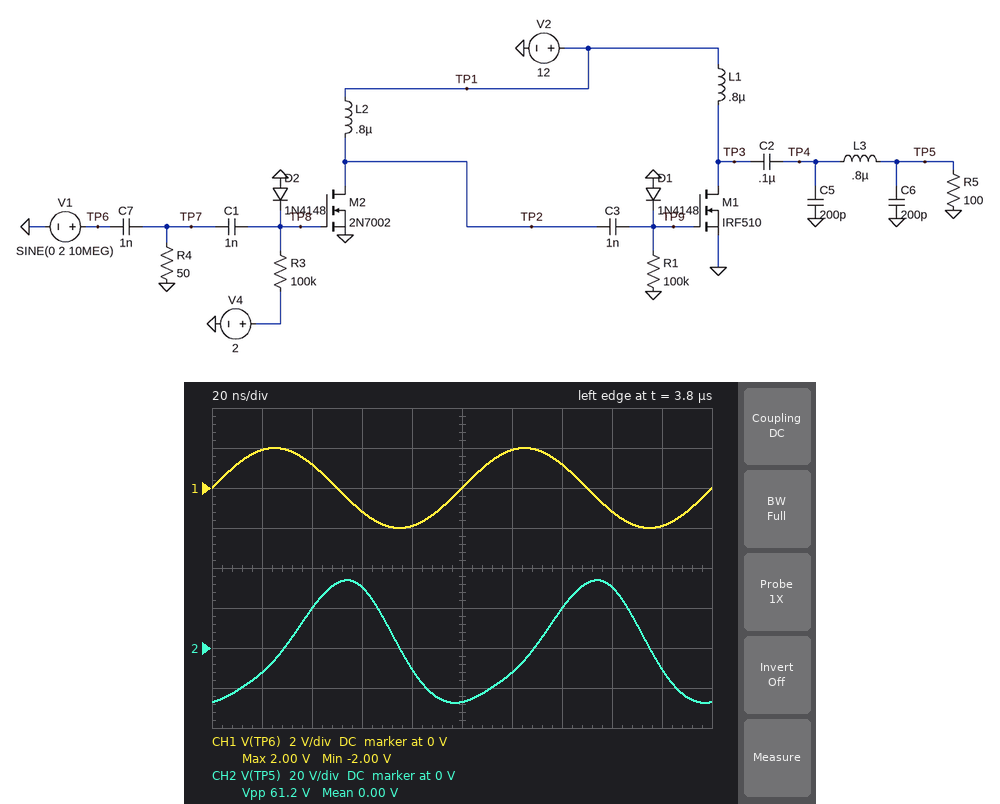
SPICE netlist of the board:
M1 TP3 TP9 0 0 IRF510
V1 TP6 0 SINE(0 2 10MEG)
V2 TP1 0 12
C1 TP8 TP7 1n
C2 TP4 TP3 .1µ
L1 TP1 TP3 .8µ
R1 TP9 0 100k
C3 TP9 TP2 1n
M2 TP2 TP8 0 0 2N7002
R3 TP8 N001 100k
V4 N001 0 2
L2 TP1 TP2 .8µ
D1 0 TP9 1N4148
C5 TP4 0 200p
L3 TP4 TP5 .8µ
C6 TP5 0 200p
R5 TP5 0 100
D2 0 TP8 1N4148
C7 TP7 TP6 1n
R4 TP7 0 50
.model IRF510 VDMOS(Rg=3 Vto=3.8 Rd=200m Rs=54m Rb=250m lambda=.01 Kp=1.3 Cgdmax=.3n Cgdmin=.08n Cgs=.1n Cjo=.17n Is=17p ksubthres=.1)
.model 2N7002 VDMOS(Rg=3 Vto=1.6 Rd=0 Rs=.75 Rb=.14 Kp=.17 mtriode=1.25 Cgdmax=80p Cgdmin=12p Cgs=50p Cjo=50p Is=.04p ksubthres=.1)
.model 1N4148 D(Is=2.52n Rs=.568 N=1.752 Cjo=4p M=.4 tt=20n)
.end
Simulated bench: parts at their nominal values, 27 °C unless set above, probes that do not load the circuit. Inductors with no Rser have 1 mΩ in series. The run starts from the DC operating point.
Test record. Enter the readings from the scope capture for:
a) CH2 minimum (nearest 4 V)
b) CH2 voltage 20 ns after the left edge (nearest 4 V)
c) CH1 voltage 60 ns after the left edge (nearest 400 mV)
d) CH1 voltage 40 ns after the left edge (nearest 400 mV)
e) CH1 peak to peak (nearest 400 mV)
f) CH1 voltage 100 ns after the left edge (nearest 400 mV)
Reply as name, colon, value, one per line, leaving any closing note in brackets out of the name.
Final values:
CH2 minimum: -28 V
CH2 voltage 20 ns after the left edge: -12 V
CH1 voltage 60 ns after the left edge: -1.2 V
CH1 voltage 40 ns after the left edge: 1.2 V
CH1 peak to peak: 4.0 V
CH1 voltage 100 ns after the left edge: 0 V
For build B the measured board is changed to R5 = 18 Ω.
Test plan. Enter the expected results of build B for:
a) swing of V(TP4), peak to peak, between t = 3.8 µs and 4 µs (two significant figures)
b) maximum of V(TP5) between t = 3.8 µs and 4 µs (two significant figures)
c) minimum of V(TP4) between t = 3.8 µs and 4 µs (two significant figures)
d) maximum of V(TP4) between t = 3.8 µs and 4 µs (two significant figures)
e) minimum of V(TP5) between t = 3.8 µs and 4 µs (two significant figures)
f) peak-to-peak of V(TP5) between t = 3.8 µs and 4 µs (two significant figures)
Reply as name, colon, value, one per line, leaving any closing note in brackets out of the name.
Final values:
swing of V(TP4), peak to peak, between t = 3.8 µs and 4 µs: 44 V
maximum of V(TP5) between t = 3.8 µs and 4 µs: 8.4 V
minimum of V(TP4) between t = 3.8 µs and 4 µs: -13 V
maximum of V(TP4) between t = 3.8 µs and 4 µs: 32 V
minimum of V(TP5) between t = 3.8 µs and 4 µs: -6.8 V
peak-to-peak of V(TP5) between t = 3.8 µs and 4 µs: 15 V
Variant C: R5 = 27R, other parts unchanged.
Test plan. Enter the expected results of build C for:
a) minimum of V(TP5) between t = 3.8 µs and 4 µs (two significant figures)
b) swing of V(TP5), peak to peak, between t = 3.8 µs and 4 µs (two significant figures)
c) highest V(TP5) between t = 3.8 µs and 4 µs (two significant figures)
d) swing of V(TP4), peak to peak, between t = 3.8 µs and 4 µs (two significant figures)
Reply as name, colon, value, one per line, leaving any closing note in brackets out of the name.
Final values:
minimum of V(TP5) between t = 3.8 µs and 4 µs: -9.3 V
swing of V(TP5), peak to peak, between t = 3.8 µs and 4 µs: 22 V
highest V(TP5) between t = 3.8 µs and 4 µs: 12 V
swing of V(TP4), peak to peak, between t = 3.8 µs and 4 µs: 43 V
